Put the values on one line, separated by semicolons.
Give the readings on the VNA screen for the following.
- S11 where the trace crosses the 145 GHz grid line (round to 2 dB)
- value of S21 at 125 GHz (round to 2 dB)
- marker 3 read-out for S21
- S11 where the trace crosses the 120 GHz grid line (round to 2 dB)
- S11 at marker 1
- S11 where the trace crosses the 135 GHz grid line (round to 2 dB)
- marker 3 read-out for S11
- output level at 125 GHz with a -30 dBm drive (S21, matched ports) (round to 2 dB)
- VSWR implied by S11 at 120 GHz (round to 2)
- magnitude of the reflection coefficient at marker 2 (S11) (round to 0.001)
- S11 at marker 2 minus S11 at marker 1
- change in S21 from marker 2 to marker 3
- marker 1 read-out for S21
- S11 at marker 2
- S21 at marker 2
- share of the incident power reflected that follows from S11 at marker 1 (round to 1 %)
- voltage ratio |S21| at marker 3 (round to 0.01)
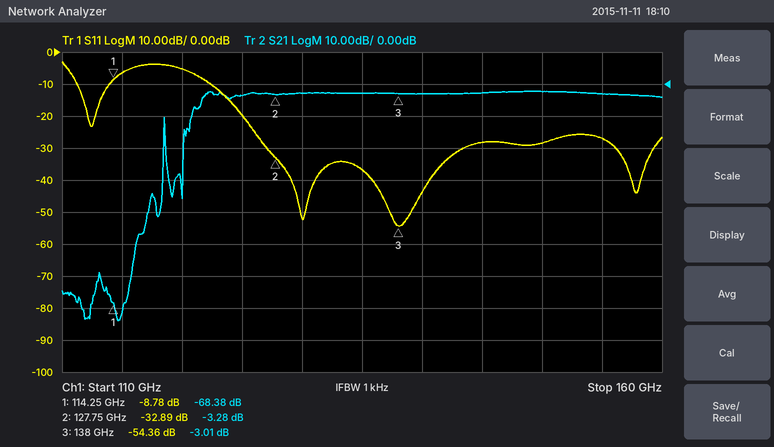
-28 dB; -4 dB; -3.01 dB; -6 dB; -8.78 dB; -36 dB; -54.36 dB; -34 dBm; 4; 0.023; -24.11 dB; 0.27 dB; -68.38 dB; -32.89 dB; -3.28 dB; 13 %; 0.71
